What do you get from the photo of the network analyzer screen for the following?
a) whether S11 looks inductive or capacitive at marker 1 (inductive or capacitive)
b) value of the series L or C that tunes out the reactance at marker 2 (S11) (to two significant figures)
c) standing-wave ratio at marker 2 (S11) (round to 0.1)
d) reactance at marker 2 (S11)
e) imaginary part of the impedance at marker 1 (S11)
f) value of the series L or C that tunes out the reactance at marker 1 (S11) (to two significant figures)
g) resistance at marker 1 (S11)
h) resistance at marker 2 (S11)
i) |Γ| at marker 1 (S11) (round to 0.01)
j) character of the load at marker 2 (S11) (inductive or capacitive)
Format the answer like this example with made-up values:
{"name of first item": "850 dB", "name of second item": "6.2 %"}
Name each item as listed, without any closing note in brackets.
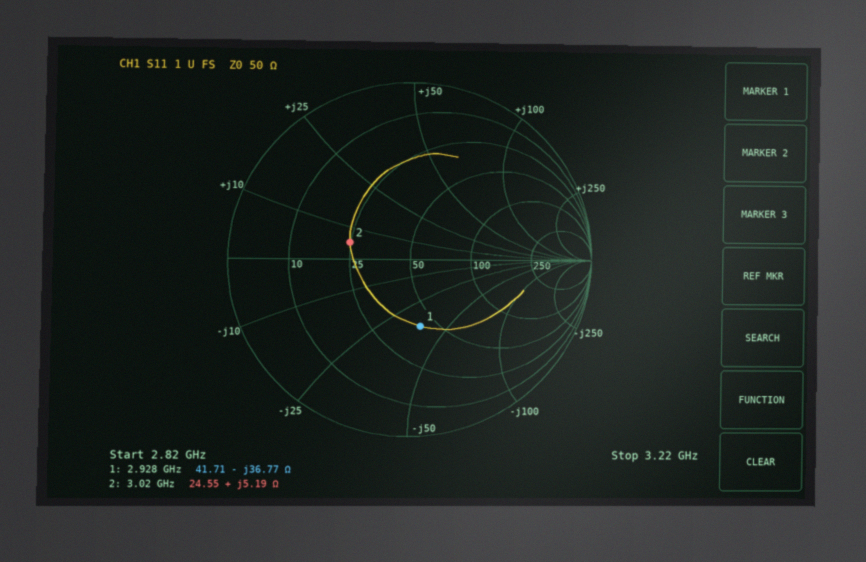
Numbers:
{"whether S11 looks inductive or capacitive at marker 1": "capacitive", "value of the series L or C that tunes out the reactance at marker 2 (S11)": "10 pF", "standing-wave ratio at marker 2 (S11)": "2.1", "reactance at marker 2": "+5.19 Ω", "imaginary part of the impedance at marker 1": "-36.77 Ω", "value of the series L or C that tunes out the reactance at marker 1 (S11)": "2.0 nH", "resistance at marker 1": "41.71 Ω", "resistance at marker 2": "24.55 Ω", "|Γ| at marker 1 (S11)": "0.38", "character of the load at marker 2 (S11)": "inductive"}
